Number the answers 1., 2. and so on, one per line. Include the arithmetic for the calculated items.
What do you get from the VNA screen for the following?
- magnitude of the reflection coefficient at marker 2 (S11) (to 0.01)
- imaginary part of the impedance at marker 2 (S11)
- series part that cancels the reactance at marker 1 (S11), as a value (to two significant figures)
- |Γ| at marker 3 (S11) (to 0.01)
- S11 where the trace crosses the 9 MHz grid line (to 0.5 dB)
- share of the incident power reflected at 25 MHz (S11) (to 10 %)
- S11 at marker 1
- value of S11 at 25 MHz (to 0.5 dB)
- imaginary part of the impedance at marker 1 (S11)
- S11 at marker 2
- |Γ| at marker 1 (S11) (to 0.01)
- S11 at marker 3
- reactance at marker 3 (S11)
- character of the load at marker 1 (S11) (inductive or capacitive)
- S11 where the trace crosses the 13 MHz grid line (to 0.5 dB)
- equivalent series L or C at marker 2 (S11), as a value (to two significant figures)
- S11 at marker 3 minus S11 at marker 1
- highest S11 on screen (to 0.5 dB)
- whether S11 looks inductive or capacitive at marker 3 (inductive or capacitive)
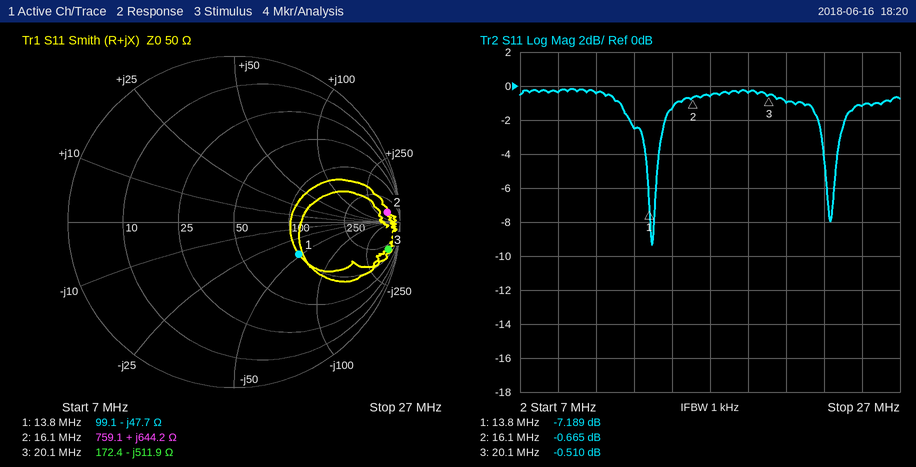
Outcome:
1. 0.93
2. +644.2 Ω
3. L = 47.7 Ω/(2π × 13.8 MHz) ≈ 550 nH
4. 0.94
5. -0.5 dB
6. 10^(-1/10) ≈ 79.4 %, so 80 % to the nearest 10 %
7. -7.189 dB
8. -1.0 dB
9. -47.7 Ω
10. -0.665 dB
11. 0.44
12. -0.510 dB
13. -511.9 Ω
14. capacitive
15. -2.5 dB
16. L = 644.2 Ω/(2π × 16.1 MHz) ≈ 6.4 µH
17. -0.51 − (-7.189) = 6.679 dB
18. 0.0 dB
19. capacitive
